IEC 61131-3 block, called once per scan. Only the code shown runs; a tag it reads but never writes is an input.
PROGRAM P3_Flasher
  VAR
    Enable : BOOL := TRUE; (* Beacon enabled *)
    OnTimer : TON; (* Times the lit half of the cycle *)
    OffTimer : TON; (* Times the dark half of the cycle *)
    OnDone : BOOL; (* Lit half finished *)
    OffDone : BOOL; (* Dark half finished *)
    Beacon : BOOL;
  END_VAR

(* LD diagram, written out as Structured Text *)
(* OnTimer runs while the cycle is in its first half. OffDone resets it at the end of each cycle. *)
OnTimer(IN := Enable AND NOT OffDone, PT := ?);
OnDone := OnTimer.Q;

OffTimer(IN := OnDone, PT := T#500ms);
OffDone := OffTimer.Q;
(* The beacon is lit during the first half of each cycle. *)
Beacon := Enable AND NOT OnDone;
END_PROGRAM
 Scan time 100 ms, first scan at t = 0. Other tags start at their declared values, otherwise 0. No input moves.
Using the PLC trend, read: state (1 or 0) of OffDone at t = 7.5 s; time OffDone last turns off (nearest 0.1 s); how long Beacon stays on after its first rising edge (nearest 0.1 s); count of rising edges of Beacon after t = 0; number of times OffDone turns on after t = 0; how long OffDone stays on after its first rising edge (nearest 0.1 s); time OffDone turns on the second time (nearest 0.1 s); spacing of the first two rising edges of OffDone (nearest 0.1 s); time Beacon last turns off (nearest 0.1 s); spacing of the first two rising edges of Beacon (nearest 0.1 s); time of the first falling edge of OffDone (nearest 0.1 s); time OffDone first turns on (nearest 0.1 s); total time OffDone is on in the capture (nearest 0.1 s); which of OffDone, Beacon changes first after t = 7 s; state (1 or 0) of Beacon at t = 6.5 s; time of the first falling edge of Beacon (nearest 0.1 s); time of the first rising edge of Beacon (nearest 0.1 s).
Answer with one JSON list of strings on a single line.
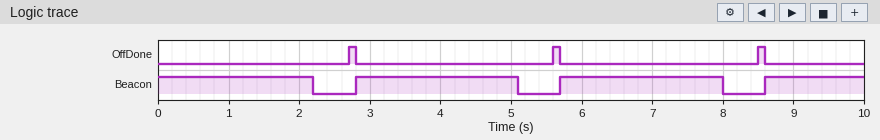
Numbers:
["0", "8.6 s", "2.3 s", "3", "3", "0.1 s", "5.6 s", "2.9 s", "8.0 s", "2.9 s", "2.8 s", "2.7 s", "0.3 s", "Beacon", "1", "2.2 s", "2.8 s"]
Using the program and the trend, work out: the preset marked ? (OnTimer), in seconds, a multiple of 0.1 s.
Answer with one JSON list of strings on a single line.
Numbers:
["2.2 s"]
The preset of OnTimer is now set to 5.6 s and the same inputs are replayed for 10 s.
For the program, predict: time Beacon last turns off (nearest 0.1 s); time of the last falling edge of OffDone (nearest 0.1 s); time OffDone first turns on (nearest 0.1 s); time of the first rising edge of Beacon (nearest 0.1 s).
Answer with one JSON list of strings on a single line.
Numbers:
["5.6 s", "6.2 s", "6.1 s", "6.2 s"]
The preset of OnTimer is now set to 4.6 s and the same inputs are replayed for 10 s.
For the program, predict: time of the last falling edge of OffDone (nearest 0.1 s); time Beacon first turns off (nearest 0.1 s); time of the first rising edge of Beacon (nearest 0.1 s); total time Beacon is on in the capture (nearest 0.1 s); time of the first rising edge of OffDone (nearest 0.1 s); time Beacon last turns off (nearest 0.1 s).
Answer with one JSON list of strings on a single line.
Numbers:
["5.2 s", "4.6 s", "5.2 s", "9.3 s", "5.1 s", "9.9 s"]
